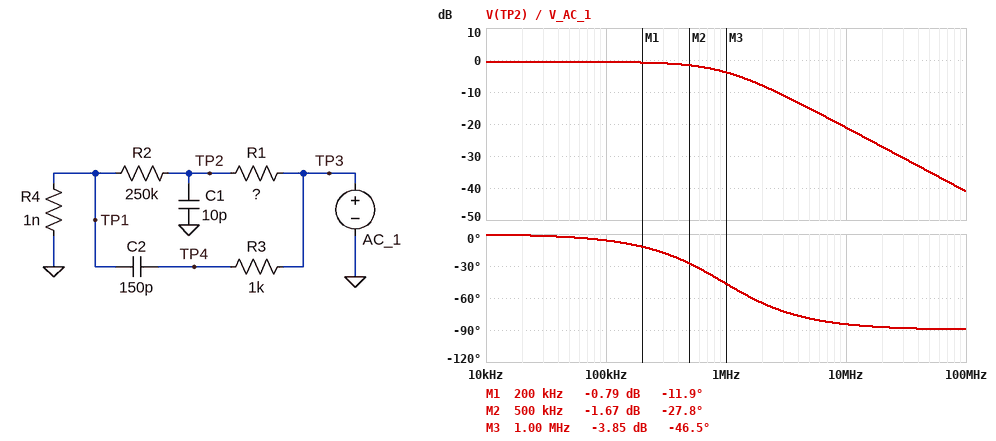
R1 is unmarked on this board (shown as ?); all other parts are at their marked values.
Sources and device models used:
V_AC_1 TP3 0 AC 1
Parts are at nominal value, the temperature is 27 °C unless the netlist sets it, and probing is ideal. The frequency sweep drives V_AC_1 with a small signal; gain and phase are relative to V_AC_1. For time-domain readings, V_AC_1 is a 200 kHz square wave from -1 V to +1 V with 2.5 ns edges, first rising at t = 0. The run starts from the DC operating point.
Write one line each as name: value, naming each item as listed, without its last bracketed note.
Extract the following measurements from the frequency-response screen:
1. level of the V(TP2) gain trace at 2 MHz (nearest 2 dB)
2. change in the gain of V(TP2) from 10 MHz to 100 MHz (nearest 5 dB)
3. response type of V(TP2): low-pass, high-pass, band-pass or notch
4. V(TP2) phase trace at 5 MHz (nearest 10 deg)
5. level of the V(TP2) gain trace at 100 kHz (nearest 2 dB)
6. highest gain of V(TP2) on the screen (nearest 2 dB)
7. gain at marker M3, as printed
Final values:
level of the V(TP2) gain trace at 2 MHz: -8 dB
change in the gain of V(TP2) from 10 MHz to 100 MHz: -20 dB
response type of V(TP2): low-pass, high-pass, band-pass or notch: low-pass
V(TP2) phase trace at 5 MHz: -80 deg
level of the V(TP2) gain trace at 100 kHz: 0 dB
highest gain of V(TP2) on the screen: 0 dB
gain at marker M3, as printed: -3.85 dB
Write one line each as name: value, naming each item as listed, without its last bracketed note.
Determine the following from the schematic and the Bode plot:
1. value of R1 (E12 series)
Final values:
value of R1: 18 kΩ
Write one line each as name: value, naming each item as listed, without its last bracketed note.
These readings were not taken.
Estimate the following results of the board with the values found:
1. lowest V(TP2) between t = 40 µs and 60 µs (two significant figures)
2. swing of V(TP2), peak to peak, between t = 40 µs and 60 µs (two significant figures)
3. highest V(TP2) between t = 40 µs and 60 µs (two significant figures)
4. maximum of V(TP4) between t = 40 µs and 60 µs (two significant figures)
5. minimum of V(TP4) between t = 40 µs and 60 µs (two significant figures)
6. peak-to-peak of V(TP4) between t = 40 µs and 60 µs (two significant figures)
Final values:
lowest V(TP2) between t = 40 µs and 60 µs: -930 mV
swing of V(TP2), peak to peak, between t = 40 µs and 60 µs: 1.9 V
highest V(TP2) between t = 40 µs and 60 µs: 930 mV
maximum of V(TP4) between t = 40 µs and 60 µs: 1.0 V
minimum of V(TP4) between t = 40 µs and 60 µs: -1.0 V
peak-to-peak of V(TP4) between t = 40 µs and 60 µs: 2.0 V
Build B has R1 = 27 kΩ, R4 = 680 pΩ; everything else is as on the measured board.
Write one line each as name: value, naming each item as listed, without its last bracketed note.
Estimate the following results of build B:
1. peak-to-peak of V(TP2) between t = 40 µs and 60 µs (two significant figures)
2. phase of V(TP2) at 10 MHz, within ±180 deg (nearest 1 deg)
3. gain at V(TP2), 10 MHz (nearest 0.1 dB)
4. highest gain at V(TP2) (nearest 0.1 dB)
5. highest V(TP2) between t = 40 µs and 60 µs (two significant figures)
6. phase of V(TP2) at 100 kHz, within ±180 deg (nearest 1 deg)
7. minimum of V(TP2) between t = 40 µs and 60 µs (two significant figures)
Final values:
peak-to-peak of V(TP2) between t = 40 µs and 60 µs: 1.8 V
phase of V(TP2) at 10 MHz, within ±180 deg: -86 deg
gain at V(TP2), 10 MHz: -24.6 dB
highest gain at V(TP2): -0.9 dB
highest V(TP2) between t = 40 µs and 60 µs: 900 mV
phase of V(TP2) at 100 kHz, within ±180 deg: -9 deg
minimum of V(TP2) between t = 40 µs and 60 µs: -900 mV
